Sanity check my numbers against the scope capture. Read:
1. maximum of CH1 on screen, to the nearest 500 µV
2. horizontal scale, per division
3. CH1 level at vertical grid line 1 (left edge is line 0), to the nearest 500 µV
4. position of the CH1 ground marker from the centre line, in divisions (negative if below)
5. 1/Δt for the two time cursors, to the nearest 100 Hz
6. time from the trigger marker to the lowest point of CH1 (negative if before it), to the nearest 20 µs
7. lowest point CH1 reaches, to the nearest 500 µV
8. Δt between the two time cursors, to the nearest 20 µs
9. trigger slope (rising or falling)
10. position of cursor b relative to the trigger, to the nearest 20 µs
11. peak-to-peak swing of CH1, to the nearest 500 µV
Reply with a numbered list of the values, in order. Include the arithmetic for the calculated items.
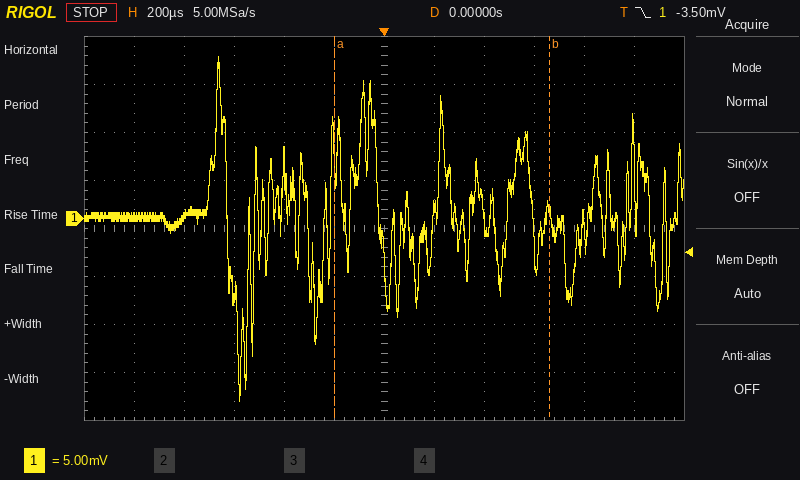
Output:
1. 17.0 mV
2. 200 µs
3. 0.0 mV
4. +0.2 div
5. 1 / 860 µs ≈ 1.2 kHz
6. -580 µs
7. -19.0 mV
8. 860 µs
9. falling
10. +660 µs
11. 17.0 mV − (-19.0 mV) = 36.0 mV
